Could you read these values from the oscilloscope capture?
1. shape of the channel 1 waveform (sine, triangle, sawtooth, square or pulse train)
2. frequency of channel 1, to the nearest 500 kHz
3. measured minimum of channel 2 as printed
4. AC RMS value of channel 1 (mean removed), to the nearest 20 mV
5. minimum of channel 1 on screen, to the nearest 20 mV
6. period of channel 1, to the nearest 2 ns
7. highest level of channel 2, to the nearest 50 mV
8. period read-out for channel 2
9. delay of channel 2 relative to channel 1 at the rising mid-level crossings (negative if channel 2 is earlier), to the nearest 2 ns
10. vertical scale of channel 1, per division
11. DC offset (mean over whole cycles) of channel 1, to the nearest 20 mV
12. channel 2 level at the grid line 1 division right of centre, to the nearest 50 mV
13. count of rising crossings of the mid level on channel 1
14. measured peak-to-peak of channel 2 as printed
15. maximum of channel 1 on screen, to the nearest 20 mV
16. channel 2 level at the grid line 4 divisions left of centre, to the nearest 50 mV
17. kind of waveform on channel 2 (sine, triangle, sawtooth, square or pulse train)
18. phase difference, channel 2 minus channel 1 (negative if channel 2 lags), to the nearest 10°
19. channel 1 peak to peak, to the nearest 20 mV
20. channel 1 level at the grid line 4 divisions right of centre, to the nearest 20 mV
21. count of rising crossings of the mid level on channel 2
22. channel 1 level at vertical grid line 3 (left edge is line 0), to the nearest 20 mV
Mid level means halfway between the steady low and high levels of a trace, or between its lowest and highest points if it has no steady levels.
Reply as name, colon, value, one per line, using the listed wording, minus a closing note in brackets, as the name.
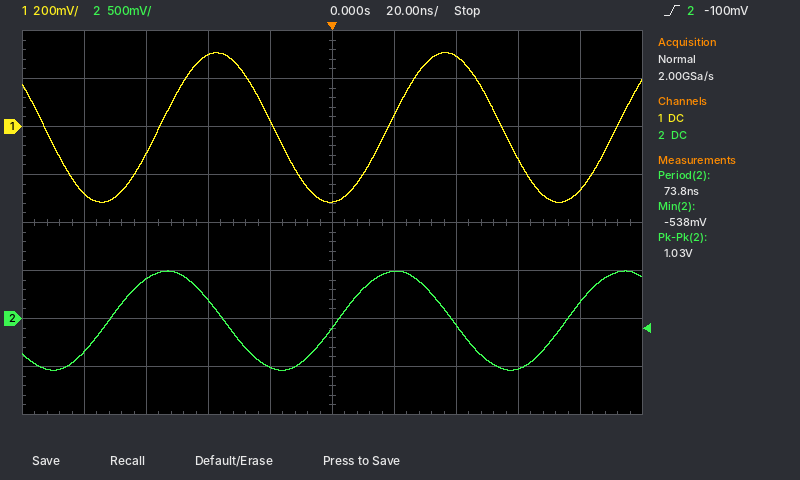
shape of the channel 1 waveform: sine
frequency of channel 1, to the nearest 500 kHz: 13.5 MHz
measured minimum of channel 2 as printed: -538 mV
AC RMS value of channel 1 (mean removed), to the nearest 20 mV: 220 mV
minimum of channel 1 on screen, to the nearest 20 mV: -320 mV
period of channel 1, to the nearest 2 ns: 74 ns
highest level of channel 2, to the nearest 50 mV: 500 mV
period read-out for channel 2: 73.8 ns
delay of channel 2 relative to channel 1 at the rising mid-level crossings (negative if channel 2 is earlier), to the nearest 2 ns: -16 ns
vertical scale of channel 1, per division: 200 mV
DC offset (mean over whole cycles) of channel 1, to the nearest 20 mV: 0 mV
channel 2 level at the grid line 1 division right of centre, to the nearest 50 mV: 500 mV
count of rising crossings of the mid level on channel 1: 3
measured peak-to-peak of channel 2 as printed: 1.03 V
maximum of channel 1 on screen, to the nearest 20 mV: 300 mV
channel 2 level at the grid line 4 divisions left of centre, to the nearest 50 mV: -350 mV
kind of waveform on channel 2: sine
phase difference, channel 2 minus channel 1 (negative if channel 2 lags), to the nearest 10°: +80°
channel 1 peak to peak, to the nearest 20 mV: 620 mV
channel 1 level at the grid line 4 divisions right of centre, to the nearest 20 mV: -260 mV
count of rising crossings of the mid level on channel 2: 3
channel 1 level at vertical grid line 3 (left edge is line 0), to the nearest 20 mV: 300 mV
